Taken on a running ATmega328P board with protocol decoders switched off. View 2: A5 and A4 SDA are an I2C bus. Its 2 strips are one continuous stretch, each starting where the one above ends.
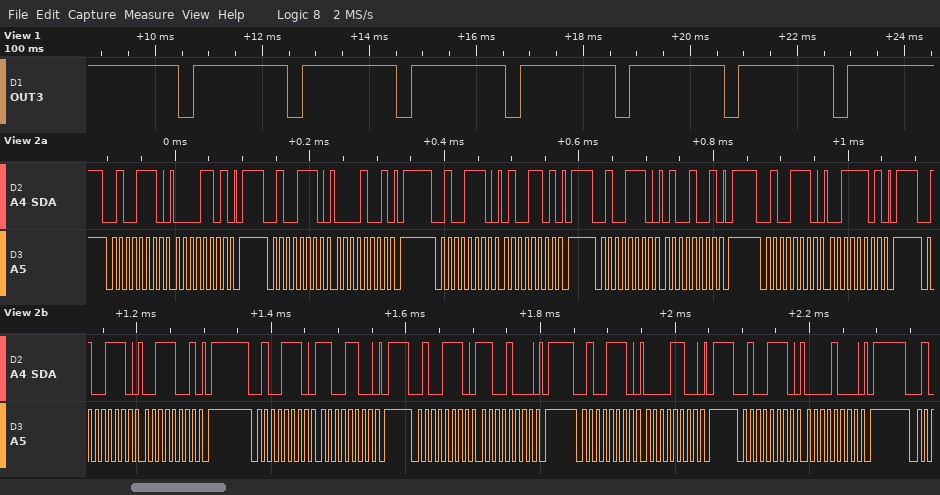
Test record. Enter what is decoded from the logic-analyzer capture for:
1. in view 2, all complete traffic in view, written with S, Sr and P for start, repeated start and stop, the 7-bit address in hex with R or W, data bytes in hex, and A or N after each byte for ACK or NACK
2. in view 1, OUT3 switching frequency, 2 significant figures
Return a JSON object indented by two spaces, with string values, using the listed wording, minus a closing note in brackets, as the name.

{
  "in view 2, all complete traffic in view, written with S, Sr and P for start, repeated start and stop, the 7-bit address in hex with R or W, data bytes in hex, and A or N after each byte for ACK or NACK": "S 27W A 0D A P S 27W A 09 A P S 27W A 4D A P S 27W A 49 A P S 27W A 3D A P S 27W A 39 A P S 27W A CC A P S 27W A C8 A P S 27W A 0C A P S 27W A 08 A P",
  "in view 1, OUT3 switching frequency, 2 significant figures": "490 Hz"
}
